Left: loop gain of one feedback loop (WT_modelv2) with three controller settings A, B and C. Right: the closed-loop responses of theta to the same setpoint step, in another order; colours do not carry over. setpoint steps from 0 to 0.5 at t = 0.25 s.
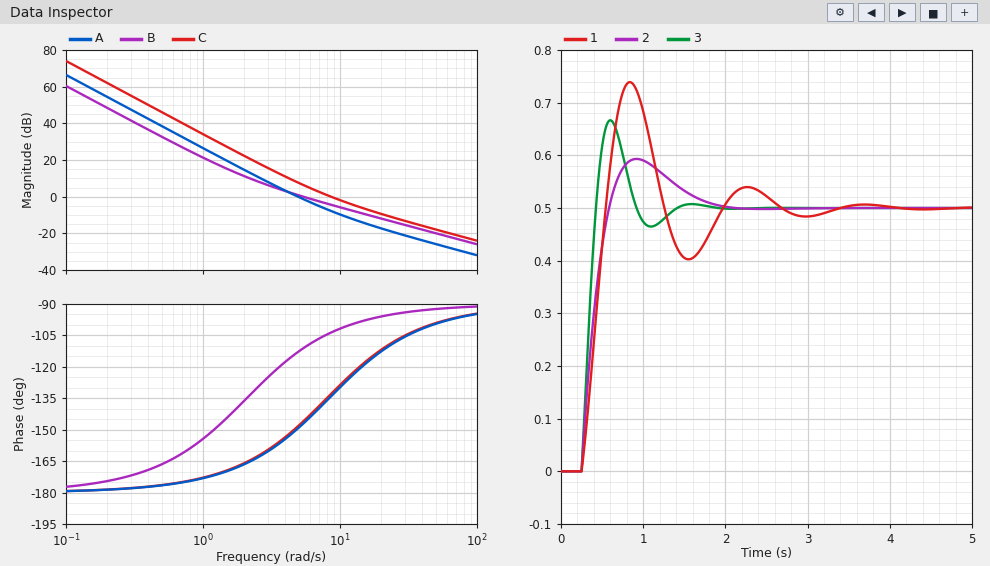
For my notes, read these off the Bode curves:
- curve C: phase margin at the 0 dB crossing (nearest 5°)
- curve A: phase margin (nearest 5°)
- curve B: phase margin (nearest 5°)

45°
30°
70°
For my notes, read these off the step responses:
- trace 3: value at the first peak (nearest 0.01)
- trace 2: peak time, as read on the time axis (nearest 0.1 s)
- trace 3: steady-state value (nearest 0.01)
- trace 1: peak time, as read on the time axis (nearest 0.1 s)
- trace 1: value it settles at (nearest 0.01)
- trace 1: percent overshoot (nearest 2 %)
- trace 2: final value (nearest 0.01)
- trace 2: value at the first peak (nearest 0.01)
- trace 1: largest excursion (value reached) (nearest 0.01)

0.67
0.9 s
0.50
0.8 s
0.50
48 %
0.50
0.59
0.74
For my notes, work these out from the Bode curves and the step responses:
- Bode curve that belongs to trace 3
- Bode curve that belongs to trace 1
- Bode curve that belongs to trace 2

C
A
B
